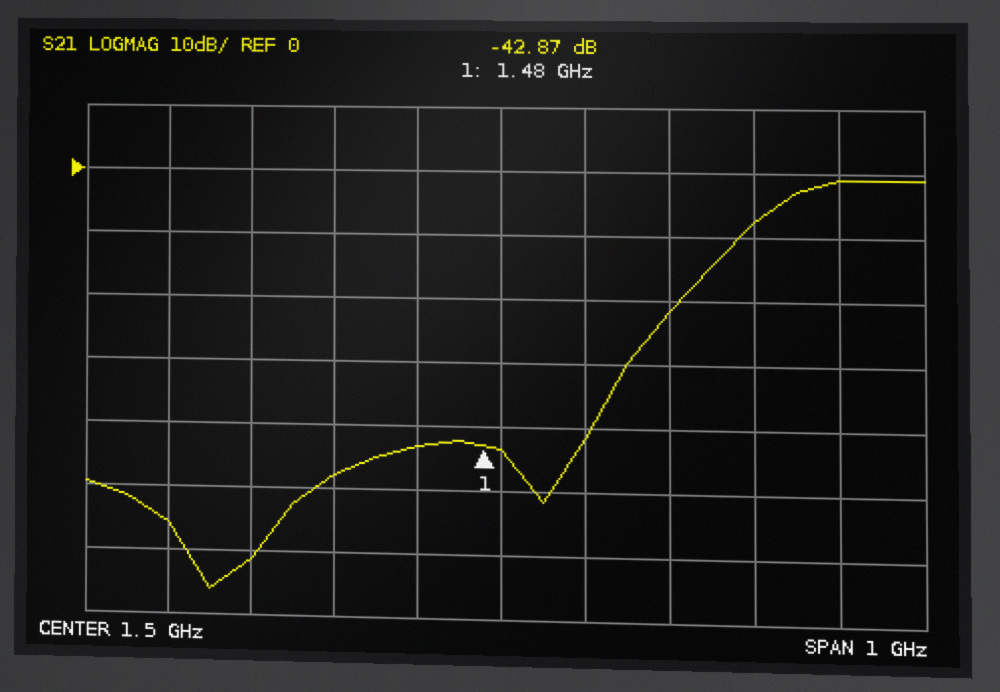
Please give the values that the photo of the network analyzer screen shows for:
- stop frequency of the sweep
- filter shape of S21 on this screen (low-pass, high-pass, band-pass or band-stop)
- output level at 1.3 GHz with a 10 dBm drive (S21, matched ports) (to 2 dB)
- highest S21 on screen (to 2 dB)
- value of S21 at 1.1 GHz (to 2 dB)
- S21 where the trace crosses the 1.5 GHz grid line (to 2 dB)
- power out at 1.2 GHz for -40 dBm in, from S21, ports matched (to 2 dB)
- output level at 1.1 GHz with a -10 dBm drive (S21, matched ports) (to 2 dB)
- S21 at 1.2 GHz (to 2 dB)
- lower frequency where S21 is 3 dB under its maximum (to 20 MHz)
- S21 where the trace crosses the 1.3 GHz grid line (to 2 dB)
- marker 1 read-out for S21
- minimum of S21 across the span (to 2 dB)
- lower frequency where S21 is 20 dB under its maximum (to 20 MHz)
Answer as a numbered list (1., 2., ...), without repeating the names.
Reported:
1. 2 GHz
2. high-pass
3. -38 dBm
4. 0 dB
5. -56 dB
6. -44 dB
7. -102 dBm
8. -66 dBm
9. -62 dB
10. 1.84 GHz
11. -48 dB
12. -42.87 dB
13. -66 dB
14. 1.70 GHz
